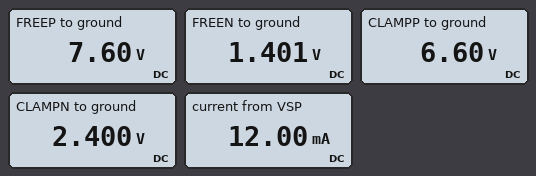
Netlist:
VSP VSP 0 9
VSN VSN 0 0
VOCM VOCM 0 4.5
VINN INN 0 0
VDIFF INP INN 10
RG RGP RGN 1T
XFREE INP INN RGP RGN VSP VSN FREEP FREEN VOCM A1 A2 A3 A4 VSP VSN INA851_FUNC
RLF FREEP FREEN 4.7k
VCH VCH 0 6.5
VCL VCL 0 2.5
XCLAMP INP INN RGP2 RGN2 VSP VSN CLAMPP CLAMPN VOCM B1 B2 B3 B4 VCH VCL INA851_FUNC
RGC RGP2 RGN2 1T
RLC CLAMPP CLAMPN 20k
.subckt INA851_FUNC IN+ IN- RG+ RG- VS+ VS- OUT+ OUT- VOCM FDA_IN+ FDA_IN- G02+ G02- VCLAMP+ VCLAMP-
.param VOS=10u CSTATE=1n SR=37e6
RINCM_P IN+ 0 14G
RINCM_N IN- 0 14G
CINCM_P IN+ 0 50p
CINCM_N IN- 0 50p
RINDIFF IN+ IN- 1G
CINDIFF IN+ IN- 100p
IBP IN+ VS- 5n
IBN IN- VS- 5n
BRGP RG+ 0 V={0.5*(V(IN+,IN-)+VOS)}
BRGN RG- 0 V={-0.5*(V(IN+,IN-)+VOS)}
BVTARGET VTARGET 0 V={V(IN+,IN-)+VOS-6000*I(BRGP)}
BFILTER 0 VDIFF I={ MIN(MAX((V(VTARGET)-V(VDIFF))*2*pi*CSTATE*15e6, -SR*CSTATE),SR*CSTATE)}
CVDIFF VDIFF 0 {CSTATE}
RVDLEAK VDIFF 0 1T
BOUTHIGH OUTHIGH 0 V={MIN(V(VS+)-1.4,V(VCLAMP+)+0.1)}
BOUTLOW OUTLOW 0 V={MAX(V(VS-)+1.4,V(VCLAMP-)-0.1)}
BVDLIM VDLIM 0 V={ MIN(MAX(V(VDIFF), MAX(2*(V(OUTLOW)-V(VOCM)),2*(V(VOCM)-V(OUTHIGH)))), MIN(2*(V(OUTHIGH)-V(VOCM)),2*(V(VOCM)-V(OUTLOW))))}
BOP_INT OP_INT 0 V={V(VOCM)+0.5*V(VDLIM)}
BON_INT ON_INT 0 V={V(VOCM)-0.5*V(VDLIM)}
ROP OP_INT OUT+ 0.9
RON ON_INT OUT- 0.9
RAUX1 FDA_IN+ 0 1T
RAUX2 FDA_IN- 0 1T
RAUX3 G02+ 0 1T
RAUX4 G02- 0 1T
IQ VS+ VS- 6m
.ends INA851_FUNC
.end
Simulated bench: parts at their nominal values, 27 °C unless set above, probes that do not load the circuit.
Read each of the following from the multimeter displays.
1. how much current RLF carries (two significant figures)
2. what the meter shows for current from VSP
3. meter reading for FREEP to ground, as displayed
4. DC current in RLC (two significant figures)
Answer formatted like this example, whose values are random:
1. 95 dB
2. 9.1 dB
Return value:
1. 1.3 mA
2. 12.00 mA
3. 7.60 V
4. 210 µA
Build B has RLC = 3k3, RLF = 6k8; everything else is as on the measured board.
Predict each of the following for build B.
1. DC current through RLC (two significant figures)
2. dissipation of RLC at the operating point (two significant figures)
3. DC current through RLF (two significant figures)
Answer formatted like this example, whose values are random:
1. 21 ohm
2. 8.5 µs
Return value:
1. 1.3 mA
2. 5.3 mW
3. 910 µA
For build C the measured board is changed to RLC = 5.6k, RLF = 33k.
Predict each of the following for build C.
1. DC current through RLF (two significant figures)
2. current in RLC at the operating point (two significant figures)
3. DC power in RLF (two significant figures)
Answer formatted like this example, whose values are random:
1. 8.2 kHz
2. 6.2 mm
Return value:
1. 190 µA
2. 750 µA
3. 1.2 mW
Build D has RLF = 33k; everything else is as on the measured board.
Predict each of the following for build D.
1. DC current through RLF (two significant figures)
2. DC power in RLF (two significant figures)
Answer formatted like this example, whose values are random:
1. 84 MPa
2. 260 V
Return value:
1. 190 µA
2. 1.2 mW
